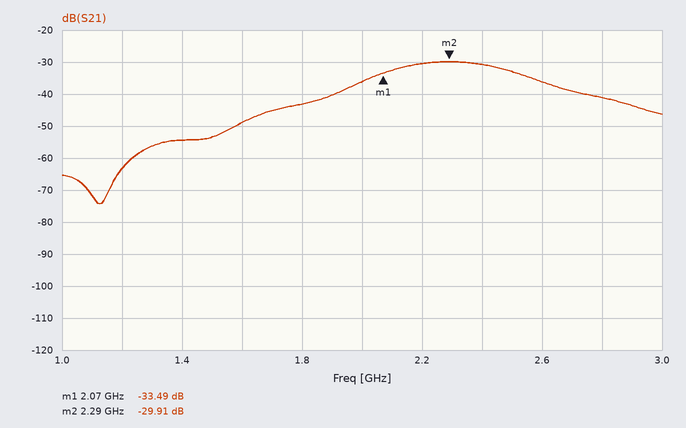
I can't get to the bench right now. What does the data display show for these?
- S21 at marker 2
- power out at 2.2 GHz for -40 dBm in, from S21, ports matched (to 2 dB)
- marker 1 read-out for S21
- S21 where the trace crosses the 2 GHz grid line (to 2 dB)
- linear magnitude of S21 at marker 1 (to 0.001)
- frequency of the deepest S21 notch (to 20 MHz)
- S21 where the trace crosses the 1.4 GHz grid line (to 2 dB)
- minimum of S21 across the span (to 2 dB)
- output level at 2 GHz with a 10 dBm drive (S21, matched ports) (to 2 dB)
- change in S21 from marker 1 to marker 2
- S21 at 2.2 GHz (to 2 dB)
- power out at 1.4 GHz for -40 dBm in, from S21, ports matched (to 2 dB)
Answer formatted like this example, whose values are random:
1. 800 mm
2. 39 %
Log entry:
1. -29.91 dB
2. -70 dBm
3. -33.49 dB
4. -36 dB
5. 0.021
6. 1.12 GHz
7. -54 dB
8. -74 dB
9. -26 dBm
10. 3.58 dB
11. -30 dB
12. -94 dBm
